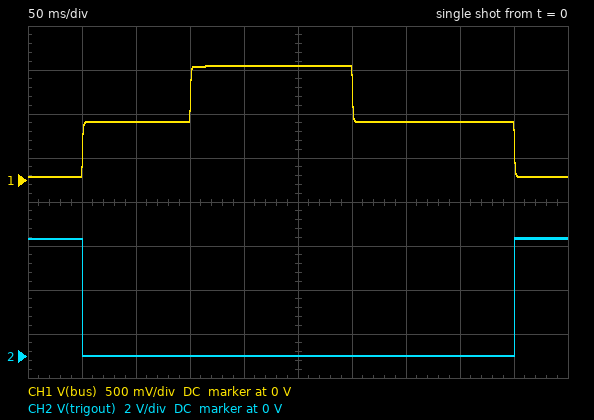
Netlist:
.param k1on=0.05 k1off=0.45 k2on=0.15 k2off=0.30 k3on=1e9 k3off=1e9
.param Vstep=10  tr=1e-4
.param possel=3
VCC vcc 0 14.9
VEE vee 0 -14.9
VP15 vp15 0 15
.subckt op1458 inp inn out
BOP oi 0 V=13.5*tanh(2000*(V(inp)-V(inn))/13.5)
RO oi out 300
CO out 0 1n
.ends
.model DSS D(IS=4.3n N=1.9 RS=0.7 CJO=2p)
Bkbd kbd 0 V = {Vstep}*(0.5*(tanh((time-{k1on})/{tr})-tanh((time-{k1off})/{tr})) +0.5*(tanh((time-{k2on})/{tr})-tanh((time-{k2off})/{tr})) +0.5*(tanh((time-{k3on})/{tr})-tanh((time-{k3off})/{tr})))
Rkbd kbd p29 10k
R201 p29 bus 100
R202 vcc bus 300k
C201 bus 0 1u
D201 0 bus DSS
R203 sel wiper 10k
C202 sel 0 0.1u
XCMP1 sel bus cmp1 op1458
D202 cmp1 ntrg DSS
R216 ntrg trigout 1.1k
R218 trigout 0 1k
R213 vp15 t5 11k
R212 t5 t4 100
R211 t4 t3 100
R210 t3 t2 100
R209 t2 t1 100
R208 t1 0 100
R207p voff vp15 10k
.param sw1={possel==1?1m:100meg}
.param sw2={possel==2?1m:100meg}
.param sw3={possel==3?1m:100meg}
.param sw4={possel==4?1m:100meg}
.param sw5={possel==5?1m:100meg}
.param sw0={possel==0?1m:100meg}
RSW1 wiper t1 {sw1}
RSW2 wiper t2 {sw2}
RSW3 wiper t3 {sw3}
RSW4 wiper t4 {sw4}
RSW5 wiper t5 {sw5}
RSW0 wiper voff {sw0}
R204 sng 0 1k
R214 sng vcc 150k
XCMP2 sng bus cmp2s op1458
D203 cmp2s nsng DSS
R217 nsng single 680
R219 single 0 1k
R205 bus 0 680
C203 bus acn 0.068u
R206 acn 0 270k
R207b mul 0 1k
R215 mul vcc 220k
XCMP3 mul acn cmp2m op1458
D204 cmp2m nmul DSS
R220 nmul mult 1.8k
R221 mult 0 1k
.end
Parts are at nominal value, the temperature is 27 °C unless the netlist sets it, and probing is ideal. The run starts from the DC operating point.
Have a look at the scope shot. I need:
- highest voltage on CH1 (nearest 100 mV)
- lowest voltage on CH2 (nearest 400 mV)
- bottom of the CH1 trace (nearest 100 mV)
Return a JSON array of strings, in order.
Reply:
["1.3 V", "0 V", "0 V"]
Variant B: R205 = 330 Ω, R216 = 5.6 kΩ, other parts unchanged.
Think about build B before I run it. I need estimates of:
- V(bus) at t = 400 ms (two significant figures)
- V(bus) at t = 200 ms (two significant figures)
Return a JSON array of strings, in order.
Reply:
["330 mV", "650 mV"]
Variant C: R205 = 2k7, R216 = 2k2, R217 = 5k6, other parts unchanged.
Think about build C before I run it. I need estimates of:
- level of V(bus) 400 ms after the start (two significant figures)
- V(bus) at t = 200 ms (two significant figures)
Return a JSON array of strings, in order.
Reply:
["2.2 V", "4.3 V"]
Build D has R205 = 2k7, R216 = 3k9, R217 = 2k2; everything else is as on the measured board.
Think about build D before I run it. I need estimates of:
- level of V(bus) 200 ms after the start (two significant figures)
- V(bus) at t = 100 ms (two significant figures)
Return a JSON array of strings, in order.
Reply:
["4.3 V", "2.2 V"]
